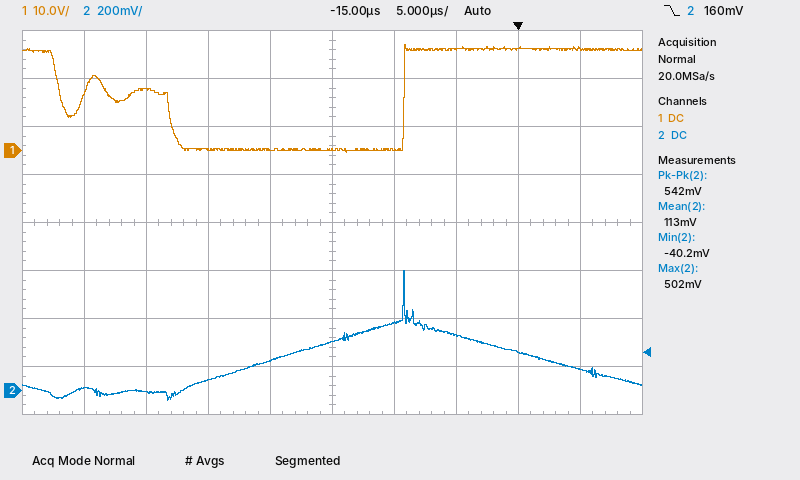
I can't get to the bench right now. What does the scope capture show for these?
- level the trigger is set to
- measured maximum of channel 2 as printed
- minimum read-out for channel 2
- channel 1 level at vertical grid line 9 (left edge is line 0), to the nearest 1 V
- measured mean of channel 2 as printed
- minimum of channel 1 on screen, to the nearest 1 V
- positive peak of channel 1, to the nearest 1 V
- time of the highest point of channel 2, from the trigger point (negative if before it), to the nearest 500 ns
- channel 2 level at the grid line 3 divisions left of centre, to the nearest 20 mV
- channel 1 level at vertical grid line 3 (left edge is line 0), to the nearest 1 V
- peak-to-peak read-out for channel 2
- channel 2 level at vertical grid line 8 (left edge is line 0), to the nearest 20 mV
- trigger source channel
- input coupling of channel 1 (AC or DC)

160 mV
502 mV
-40.2 mV
21 V
113 mV
0 V
22 V
-9.0 µs
0 mV
0 V
542 mV
160 mV
channel 2
DC
